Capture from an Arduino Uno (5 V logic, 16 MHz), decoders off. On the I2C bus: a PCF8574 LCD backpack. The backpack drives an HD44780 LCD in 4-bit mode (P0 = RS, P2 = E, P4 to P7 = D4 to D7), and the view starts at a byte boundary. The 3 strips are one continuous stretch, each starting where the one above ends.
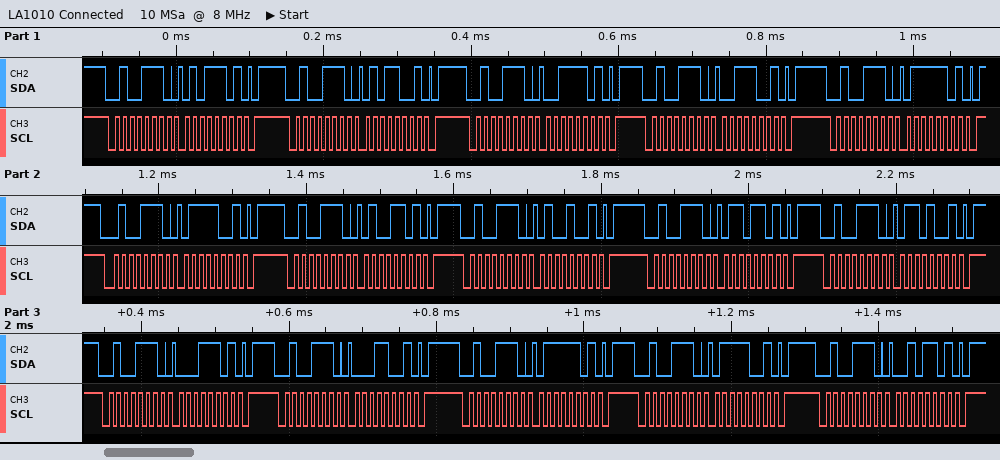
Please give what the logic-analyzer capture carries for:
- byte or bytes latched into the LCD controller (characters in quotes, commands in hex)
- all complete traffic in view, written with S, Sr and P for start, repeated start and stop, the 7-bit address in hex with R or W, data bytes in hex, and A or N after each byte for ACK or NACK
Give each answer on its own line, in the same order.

'S' 't' 'a'
S 27W A 5D A P S 27W A 59 A P S 27W A 3D A P S 27W A 39 A P S 27W A 7D A P S 27W A 79 A P S 27W A 4D A P S 27W A 49 A P S 27W A 6D A P S 27W A 69 A P S 27W A 1D A P S 27W A 19 A P S 27W A 7D A P S 27W A 79 A P S 27W A 2D A P
